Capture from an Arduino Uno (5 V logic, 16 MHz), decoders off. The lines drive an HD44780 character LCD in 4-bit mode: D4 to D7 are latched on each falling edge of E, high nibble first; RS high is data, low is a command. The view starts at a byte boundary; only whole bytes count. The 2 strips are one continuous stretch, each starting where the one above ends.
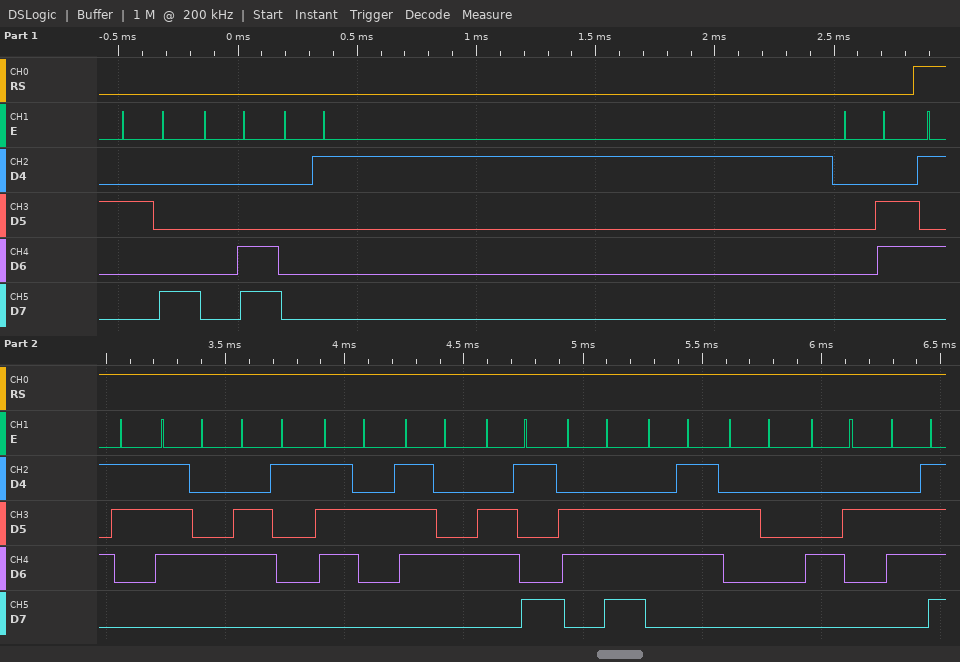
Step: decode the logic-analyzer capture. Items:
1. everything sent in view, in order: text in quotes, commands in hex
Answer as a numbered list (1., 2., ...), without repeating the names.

1. 0x28 0x0C 0x01 0x06 "Starting Bo"
